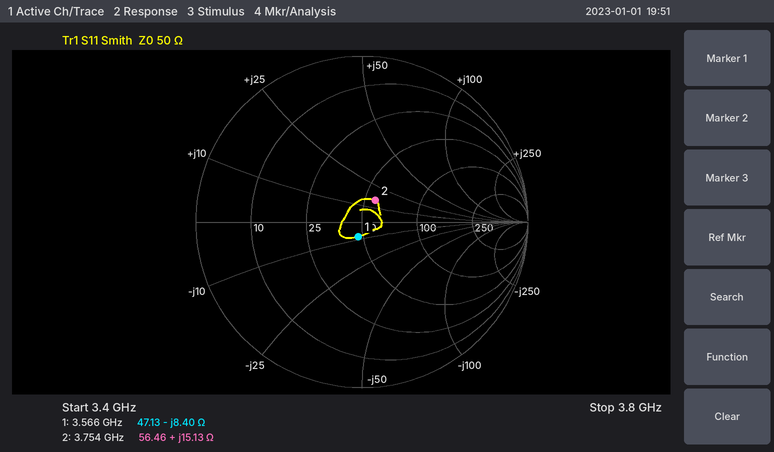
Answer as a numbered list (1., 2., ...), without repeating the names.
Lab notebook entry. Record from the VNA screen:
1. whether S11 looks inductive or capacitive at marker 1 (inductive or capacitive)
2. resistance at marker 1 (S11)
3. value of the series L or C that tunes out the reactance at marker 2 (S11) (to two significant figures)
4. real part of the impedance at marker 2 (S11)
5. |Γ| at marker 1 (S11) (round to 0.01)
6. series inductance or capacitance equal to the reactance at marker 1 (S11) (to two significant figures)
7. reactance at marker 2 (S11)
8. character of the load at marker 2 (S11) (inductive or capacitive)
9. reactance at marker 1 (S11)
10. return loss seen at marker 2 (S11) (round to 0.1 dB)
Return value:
1. capacitive
2. 47.13 Ω
3. 2.8 pF
4. 56.46 Ω
5. 0.09
6. 5.3 pF
7. +15.13 Ω
8. inductive
9. -8.40 Ω
10. 16.3 dB
